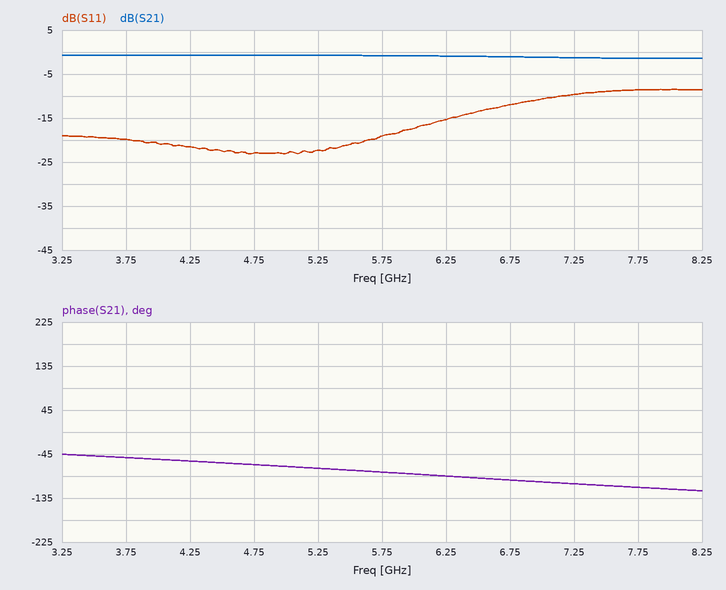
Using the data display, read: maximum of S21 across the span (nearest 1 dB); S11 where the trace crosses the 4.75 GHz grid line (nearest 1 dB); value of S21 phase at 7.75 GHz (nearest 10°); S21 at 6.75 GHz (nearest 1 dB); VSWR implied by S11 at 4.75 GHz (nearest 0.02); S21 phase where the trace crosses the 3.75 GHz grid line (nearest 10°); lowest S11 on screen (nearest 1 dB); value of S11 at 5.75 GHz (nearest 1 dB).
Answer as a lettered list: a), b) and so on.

a) -1 dB
b) -23 dB
c) -110°
d) -1 dB
e) 1.16
f) -50°
g) -23 dB
h) -19 dB
